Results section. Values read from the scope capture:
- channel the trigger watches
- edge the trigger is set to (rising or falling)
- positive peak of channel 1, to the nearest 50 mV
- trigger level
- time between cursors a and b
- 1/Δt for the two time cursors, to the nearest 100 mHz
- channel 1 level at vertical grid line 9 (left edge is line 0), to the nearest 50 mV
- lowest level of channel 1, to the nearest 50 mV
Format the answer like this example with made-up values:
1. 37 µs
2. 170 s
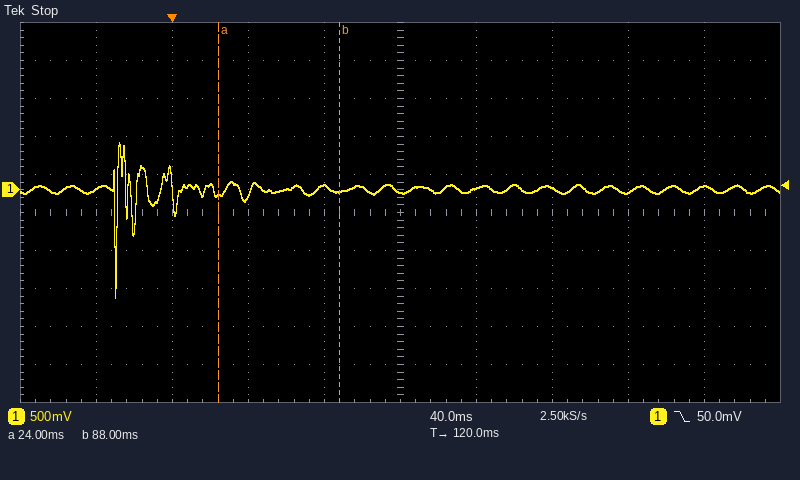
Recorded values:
1. channel 1
2. falling
3. 600 mV
4. 50.0 mV
5. 64 ms
6. 15.6 Hz
7. 50 mV
8. -1.40 V
